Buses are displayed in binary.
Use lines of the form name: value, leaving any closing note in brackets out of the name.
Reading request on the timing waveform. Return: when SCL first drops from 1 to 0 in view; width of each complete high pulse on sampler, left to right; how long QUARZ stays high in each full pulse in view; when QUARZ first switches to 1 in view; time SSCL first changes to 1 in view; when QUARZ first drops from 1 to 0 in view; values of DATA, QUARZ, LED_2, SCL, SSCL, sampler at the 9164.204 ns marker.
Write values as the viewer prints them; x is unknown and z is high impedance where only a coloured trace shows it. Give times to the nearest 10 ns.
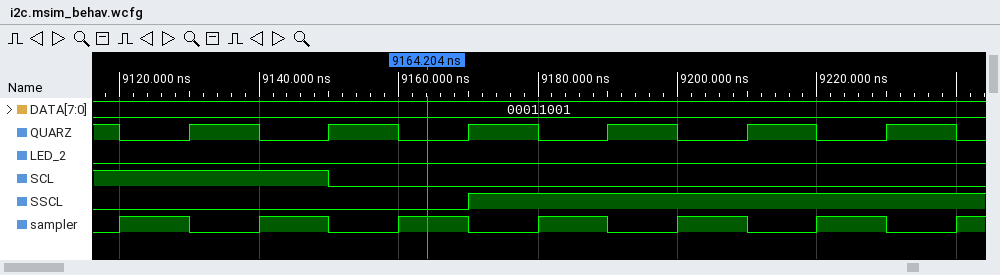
when SCL first drops from 1 to 0 in view: 9150 ns
width of each complete high pulse on sampler, left to right: 10 ns, 10 ns, 10 ns, 10 ns, 10 ns, 10 ns
how long QUARZ stays high in each full pulse in view: 10 ns, 10 ns, 10 ns, 10 ns, 10 ns, 10 ns
when QUARZ first switches to 1 in view: 9130 ns
time SSCL first changes to 1 in view: 9170 ns
when QUARZ first drops from 1 to 0 in view: 9120 ns
values of DATA, QUARZ, LED_2, SCL, SSCL, sampler at the 9164.204 ns marker: DATA=00011001, QUARZ=0, LED_2=0, SCL=0, SSCL=0, sampler=1
